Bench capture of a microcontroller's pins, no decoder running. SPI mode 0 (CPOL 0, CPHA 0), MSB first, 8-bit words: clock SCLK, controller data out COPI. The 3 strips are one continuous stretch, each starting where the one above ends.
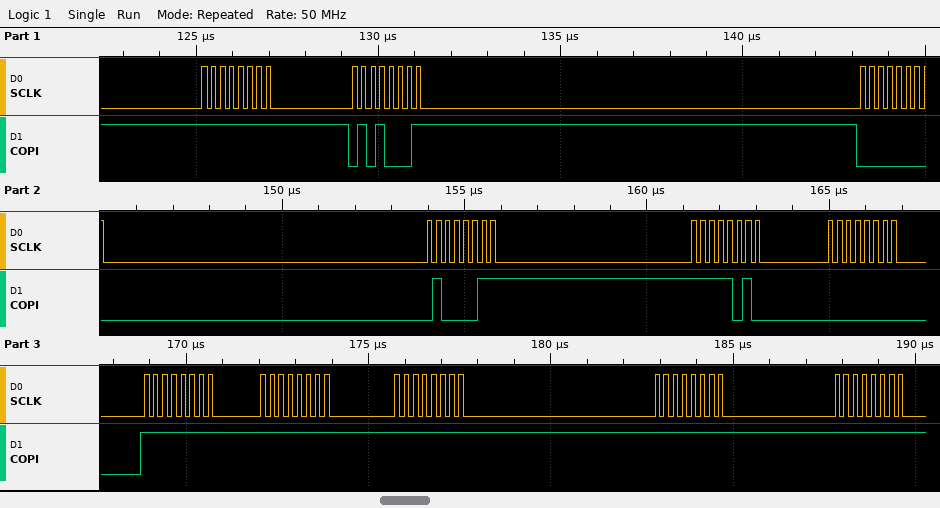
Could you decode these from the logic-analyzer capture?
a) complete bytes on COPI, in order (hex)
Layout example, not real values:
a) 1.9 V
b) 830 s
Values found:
a) 0xFF 0x51 0x00 0x43 0xFA 0x00 0xFF 0xFF 0xFF 0xFF 0xFF
